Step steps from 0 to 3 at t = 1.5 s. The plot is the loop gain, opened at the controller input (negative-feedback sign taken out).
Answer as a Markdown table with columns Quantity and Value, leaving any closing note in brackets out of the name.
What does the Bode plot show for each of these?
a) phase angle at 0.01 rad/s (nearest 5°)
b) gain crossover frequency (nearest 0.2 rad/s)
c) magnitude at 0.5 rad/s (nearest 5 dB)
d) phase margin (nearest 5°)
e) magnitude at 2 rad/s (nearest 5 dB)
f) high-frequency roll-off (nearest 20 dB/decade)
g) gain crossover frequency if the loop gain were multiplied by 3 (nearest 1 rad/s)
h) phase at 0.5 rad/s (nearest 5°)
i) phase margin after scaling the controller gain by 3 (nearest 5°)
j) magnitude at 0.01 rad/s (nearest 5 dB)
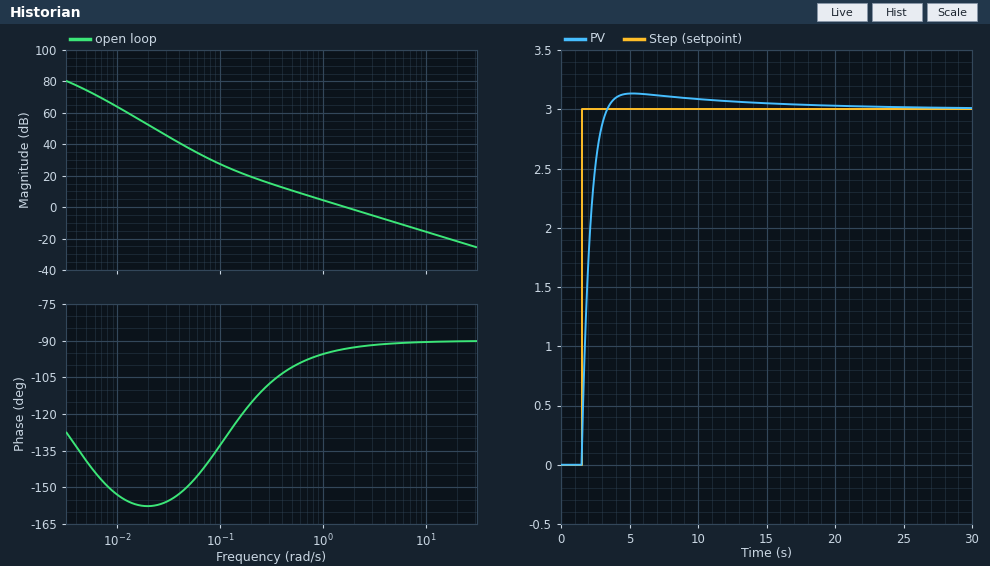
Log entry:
| Quantity | Value |
|---|---|
| phase angle at 0.01 rad/s | -155° |
| gain crossover frequency | 1.6 rad/s |
| magnitude at 0.5 rad/s | 10 dB |
| phase margin | 85° |
| magnitude at 2 rad/s | 0 dB |
| high-frequency roll-off | -20 dB/decade |
| gain crossover frequency if the loop gain were multiplied by 3 | 5 rad/s |
| phase at 0.5 rad/s | -100° |
| phase margin after scaling the controller gain by 3 | 90° |
| magnitude at 0.01 rad/s | 65 dB |
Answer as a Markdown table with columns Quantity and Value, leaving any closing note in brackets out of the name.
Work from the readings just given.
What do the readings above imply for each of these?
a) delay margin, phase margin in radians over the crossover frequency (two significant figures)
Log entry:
| Quantity | Value |
|---|---|
| delay margin, phase margin in radians over the crossover frequency | 0.93 s |
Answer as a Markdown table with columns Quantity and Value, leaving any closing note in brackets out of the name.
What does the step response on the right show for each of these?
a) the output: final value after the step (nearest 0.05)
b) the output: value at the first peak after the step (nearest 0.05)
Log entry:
| Quantity | Value |
|---|---|
| the output: final value after the step | 3.00 |
| the output: value at the first peak after the step | 3.15 |
